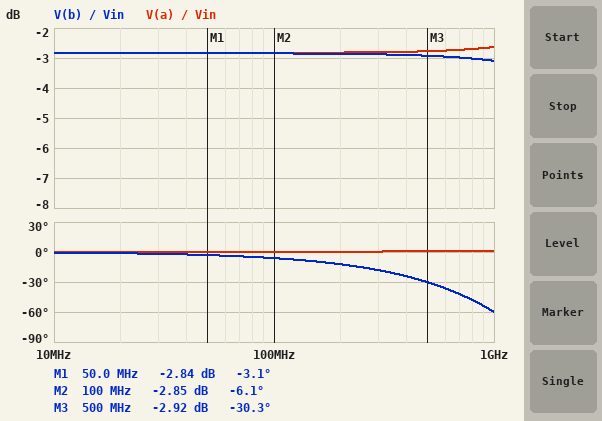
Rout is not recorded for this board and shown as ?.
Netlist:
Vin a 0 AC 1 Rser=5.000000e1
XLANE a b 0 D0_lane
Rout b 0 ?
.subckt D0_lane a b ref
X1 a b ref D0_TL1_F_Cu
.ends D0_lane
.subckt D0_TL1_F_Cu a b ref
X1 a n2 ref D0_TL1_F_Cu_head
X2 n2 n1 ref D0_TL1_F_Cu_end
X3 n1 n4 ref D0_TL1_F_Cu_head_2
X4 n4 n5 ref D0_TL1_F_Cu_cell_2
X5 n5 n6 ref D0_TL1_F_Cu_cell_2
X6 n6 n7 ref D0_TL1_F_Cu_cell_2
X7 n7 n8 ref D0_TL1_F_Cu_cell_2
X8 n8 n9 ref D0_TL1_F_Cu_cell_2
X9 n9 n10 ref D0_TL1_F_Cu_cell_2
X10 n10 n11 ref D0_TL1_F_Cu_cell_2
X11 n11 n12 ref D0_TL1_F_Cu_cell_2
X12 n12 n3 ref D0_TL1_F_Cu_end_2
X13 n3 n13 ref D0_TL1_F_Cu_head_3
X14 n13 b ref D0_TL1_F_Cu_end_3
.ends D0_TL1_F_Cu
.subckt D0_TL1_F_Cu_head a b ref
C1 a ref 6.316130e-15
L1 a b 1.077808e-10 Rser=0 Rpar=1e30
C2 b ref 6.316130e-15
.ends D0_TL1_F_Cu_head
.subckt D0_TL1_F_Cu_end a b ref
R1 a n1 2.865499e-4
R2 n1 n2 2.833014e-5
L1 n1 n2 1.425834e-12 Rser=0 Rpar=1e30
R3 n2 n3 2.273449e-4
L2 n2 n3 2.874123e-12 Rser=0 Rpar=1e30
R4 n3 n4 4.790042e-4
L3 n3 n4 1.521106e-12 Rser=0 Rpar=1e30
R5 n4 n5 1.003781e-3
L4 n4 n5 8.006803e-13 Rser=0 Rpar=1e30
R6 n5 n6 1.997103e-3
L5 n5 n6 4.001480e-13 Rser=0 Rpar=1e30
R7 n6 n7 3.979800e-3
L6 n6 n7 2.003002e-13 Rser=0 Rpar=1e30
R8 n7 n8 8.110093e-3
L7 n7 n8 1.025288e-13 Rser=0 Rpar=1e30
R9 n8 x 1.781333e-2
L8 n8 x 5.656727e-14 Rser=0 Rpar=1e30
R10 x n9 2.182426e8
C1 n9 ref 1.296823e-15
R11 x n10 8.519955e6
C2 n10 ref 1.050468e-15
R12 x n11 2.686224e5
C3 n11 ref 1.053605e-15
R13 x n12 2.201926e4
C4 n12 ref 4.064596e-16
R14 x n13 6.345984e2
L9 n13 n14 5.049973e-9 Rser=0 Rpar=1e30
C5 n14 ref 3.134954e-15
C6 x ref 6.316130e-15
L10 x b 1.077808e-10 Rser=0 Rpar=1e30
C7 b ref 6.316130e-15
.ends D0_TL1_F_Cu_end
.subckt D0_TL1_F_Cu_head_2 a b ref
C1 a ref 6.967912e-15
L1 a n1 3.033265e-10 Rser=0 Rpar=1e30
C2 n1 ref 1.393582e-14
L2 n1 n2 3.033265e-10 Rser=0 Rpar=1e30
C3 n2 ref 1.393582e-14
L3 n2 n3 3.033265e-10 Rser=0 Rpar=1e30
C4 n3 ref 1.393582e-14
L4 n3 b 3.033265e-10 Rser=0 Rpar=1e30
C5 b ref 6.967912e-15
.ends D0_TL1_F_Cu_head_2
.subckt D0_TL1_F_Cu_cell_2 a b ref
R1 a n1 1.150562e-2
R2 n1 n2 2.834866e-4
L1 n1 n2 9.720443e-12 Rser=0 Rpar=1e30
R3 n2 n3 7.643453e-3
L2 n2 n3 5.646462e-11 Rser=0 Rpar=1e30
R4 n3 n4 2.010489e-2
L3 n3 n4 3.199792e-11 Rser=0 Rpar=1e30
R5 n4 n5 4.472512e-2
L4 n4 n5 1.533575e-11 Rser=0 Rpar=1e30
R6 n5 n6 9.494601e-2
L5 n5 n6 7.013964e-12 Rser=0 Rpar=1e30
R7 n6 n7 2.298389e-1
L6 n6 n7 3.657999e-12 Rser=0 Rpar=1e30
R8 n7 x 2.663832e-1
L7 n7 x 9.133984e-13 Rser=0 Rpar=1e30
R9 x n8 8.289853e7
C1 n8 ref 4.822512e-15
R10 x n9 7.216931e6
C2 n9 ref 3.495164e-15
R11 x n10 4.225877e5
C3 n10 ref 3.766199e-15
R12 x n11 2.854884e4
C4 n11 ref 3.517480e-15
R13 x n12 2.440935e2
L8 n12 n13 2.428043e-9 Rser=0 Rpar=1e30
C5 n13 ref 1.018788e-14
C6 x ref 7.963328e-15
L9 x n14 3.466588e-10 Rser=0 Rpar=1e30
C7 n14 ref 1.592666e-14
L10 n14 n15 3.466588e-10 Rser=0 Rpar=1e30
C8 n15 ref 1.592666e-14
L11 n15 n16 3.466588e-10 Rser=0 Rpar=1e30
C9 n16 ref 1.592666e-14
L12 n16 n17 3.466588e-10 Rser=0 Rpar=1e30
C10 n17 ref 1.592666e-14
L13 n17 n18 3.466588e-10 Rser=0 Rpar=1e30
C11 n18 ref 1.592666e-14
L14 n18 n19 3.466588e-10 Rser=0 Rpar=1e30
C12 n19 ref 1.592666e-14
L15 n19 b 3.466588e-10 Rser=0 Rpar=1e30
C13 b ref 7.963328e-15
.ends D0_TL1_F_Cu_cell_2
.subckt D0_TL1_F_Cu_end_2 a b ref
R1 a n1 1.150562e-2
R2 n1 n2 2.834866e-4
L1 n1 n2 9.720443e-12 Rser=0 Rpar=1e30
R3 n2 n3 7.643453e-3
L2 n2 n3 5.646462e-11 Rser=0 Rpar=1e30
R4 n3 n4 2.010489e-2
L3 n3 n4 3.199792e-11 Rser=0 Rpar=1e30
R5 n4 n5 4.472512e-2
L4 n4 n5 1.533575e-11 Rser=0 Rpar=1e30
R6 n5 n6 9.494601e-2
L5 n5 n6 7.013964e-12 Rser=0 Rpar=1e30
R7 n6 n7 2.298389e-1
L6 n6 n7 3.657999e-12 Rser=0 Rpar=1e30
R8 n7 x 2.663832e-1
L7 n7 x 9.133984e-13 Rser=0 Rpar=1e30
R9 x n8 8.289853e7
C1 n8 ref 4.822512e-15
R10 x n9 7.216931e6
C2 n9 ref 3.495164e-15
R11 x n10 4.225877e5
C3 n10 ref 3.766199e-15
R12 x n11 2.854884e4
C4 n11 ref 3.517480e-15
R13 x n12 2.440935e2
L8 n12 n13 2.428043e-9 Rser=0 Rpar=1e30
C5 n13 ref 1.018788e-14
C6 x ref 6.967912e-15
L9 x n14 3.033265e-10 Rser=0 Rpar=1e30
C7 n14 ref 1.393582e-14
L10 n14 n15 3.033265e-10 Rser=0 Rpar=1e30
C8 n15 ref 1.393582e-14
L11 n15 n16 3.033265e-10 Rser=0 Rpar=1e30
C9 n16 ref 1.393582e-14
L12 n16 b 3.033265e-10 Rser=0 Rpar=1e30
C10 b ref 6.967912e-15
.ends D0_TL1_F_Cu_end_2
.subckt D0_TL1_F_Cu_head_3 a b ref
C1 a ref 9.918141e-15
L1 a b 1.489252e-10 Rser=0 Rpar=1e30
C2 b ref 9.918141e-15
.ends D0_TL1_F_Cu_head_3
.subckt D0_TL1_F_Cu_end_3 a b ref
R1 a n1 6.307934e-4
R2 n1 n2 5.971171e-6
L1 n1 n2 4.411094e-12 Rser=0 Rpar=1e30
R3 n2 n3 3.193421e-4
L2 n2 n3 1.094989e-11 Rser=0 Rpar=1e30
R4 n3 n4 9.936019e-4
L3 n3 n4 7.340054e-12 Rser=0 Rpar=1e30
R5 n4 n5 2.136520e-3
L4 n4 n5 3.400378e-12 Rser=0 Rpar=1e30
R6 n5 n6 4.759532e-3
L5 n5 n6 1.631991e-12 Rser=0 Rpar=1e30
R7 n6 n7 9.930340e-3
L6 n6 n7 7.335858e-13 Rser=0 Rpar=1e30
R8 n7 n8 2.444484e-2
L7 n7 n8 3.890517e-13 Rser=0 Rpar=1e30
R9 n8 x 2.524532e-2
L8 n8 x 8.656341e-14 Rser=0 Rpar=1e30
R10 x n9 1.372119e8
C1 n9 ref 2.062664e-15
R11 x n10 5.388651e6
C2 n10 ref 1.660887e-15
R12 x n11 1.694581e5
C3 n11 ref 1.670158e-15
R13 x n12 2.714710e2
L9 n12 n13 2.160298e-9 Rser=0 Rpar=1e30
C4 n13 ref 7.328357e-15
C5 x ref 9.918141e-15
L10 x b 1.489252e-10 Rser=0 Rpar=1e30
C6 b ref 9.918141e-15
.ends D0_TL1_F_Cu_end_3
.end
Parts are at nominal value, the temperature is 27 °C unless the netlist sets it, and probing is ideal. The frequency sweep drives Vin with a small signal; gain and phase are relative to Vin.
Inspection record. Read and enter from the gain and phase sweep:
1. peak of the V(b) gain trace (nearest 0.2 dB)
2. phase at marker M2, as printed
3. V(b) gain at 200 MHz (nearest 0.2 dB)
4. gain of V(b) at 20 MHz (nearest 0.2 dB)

-2.8 dB
-6.1 deg
-2.8 dB
-2.8 dB
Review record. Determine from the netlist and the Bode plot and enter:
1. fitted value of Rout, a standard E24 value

130 Ω
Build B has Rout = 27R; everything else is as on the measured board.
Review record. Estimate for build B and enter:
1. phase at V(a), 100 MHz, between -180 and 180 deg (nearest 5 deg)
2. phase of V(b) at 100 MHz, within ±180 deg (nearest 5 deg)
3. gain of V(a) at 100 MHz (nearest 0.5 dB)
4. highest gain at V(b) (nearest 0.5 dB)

15 deg
-10 deg
-8.0 dB
-9.0 dB
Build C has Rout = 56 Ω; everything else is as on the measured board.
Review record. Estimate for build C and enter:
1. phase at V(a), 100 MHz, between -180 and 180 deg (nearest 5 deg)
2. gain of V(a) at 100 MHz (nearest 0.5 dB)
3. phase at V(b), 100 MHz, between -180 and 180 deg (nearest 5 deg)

5 deg
-5.5 dB
-10 deg
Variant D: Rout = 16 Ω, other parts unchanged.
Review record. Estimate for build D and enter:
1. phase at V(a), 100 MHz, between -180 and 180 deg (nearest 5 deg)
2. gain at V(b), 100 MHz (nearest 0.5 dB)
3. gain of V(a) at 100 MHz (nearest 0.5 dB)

30 deg
-12.5 dB
-10.0 dB
